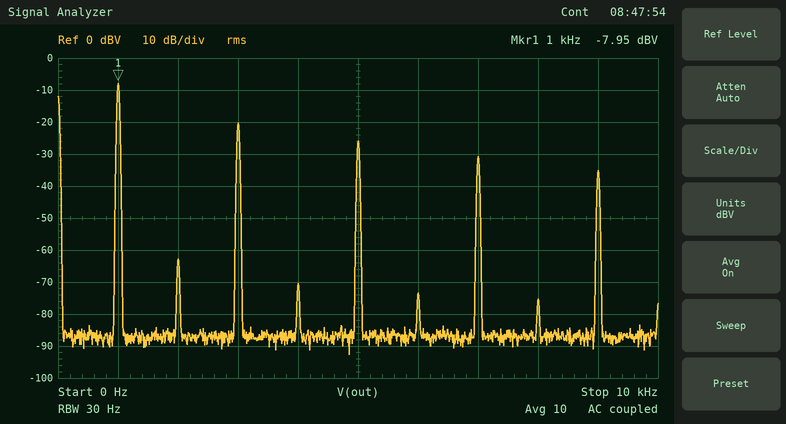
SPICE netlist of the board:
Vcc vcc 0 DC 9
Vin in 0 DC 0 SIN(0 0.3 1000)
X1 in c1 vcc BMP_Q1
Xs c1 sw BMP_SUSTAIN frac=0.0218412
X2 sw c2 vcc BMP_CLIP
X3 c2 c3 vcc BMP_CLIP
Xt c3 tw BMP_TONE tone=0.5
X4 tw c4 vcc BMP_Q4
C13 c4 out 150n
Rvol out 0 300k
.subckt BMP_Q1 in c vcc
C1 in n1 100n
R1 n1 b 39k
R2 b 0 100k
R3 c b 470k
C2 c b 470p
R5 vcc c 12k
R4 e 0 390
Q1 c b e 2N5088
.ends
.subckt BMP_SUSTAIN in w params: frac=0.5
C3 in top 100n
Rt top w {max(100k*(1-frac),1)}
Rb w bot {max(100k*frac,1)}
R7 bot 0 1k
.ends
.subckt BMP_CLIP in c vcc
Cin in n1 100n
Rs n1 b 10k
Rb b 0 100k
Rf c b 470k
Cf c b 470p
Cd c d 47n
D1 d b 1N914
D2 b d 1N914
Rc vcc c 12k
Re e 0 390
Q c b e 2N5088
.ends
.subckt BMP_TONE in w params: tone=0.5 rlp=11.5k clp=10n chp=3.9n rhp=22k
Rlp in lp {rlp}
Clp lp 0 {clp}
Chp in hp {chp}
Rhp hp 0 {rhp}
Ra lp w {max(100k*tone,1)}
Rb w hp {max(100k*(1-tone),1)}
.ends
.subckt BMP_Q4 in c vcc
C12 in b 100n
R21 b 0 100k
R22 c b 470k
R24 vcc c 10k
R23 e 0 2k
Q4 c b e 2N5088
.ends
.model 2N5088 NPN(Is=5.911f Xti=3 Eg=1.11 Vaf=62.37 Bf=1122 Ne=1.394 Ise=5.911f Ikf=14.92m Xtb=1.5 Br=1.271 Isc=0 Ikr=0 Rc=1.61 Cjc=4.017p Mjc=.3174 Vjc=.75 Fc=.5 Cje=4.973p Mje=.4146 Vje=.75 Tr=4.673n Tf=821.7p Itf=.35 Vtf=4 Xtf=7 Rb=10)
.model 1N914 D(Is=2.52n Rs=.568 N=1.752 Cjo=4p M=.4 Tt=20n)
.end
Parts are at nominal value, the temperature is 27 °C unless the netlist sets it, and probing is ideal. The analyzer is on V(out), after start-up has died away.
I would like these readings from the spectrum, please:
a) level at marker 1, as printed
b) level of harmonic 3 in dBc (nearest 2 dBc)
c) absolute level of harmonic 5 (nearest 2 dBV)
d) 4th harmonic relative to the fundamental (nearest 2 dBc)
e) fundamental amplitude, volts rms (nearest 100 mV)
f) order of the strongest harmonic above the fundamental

-7.95 dBV
-12 dBc
-26 dBV
-62 dBc
400 mV
3
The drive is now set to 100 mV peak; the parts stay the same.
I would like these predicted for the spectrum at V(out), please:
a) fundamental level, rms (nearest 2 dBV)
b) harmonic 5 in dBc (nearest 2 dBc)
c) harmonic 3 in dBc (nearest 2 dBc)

-10 dBV
-22 dBc
-14 dBc
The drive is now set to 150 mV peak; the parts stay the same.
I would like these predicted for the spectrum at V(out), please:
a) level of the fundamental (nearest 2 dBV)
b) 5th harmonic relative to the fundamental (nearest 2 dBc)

-8 dBV
-20 dBc
